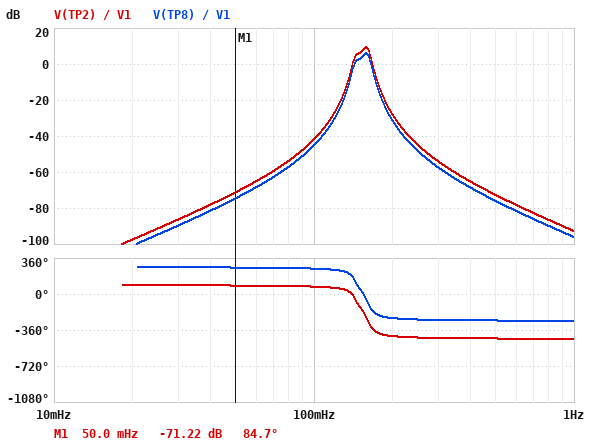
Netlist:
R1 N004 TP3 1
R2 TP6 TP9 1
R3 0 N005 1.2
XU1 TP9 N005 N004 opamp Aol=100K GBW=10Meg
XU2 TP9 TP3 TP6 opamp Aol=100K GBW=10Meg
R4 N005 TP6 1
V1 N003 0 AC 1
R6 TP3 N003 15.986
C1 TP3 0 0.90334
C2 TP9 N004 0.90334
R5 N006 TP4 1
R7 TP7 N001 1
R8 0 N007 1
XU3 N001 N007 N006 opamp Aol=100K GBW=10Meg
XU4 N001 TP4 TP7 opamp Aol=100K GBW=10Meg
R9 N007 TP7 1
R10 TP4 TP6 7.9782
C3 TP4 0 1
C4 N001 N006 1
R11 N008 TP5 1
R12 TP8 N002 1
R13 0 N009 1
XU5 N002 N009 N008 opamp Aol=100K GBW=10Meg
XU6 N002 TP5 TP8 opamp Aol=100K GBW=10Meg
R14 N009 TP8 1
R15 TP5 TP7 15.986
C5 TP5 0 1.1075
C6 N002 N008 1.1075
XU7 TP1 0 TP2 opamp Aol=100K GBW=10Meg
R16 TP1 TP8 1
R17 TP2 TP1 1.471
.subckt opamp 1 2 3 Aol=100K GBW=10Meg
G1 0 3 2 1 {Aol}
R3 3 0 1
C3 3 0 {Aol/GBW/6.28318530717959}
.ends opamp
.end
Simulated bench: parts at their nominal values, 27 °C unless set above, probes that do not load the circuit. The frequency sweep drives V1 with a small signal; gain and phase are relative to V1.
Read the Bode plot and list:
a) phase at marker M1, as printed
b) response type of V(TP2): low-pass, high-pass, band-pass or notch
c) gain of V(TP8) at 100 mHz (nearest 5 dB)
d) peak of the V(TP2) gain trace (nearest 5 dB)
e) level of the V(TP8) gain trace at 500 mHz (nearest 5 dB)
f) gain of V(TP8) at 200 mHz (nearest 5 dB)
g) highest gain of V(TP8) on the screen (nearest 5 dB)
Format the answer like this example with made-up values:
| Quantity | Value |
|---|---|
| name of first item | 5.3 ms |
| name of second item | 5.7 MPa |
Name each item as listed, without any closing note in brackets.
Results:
| Quantity | Value |
|---|---|
| phase at marker M1, as printed | 84.7 deg |
| response type of V(TP2): low-pass, high-pass, band-pass or notch | band-pass |
| gain of V(TP8) at 100 mHz | -45 dB |
| peak of the V(TP2) gain trace | 10 dB |
| level of the V(TP8) gain trace at 500 mHz | -75 dB |
| gain of V(TP8) at 200 mHz | -30 dB |
| highest gain of V(TP8) on the screen | 5 dB |
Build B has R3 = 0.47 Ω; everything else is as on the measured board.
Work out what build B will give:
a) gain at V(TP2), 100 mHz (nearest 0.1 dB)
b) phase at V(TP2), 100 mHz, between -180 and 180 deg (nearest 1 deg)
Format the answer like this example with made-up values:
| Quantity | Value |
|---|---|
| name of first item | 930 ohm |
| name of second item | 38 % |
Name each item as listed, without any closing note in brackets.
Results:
| Quantity | Value |
|---|---|
| gain at V(TP2), 100 mHz | -48.1 dB |
| phase at V(TP2), 100 mHz, between -180 and 180 deg | 77 deg |
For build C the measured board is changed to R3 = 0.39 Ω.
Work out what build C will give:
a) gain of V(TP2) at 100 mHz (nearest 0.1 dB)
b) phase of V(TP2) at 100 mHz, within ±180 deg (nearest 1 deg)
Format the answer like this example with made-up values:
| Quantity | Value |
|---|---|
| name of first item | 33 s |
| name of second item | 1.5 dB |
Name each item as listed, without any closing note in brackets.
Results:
| Quantity | Value |
|---|---|
| gain of V(TP2) at 100 mHz | -48.9 dB |
| phase of V(TP2) at 100 mHz, within ±180 deg | 77 deg |
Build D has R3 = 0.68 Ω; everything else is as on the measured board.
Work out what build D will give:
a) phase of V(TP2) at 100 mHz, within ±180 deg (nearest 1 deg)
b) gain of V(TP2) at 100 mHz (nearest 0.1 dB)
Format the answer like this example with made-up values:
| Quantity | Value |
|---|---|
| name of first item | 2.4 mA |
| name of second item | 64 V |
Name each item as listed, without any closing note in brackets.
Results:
| Quantity | Value |
|---|---|
| phase of V(TP2) at 100 mHz, within ±180 deg | 76 deg |
| gain of V(TP2) at 100 mHz | -46.2 dB |
